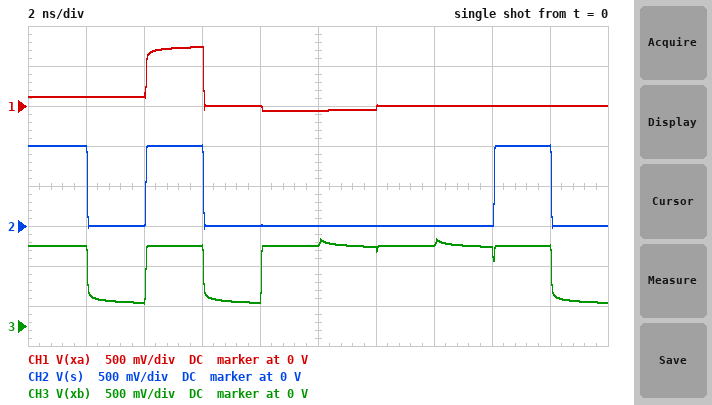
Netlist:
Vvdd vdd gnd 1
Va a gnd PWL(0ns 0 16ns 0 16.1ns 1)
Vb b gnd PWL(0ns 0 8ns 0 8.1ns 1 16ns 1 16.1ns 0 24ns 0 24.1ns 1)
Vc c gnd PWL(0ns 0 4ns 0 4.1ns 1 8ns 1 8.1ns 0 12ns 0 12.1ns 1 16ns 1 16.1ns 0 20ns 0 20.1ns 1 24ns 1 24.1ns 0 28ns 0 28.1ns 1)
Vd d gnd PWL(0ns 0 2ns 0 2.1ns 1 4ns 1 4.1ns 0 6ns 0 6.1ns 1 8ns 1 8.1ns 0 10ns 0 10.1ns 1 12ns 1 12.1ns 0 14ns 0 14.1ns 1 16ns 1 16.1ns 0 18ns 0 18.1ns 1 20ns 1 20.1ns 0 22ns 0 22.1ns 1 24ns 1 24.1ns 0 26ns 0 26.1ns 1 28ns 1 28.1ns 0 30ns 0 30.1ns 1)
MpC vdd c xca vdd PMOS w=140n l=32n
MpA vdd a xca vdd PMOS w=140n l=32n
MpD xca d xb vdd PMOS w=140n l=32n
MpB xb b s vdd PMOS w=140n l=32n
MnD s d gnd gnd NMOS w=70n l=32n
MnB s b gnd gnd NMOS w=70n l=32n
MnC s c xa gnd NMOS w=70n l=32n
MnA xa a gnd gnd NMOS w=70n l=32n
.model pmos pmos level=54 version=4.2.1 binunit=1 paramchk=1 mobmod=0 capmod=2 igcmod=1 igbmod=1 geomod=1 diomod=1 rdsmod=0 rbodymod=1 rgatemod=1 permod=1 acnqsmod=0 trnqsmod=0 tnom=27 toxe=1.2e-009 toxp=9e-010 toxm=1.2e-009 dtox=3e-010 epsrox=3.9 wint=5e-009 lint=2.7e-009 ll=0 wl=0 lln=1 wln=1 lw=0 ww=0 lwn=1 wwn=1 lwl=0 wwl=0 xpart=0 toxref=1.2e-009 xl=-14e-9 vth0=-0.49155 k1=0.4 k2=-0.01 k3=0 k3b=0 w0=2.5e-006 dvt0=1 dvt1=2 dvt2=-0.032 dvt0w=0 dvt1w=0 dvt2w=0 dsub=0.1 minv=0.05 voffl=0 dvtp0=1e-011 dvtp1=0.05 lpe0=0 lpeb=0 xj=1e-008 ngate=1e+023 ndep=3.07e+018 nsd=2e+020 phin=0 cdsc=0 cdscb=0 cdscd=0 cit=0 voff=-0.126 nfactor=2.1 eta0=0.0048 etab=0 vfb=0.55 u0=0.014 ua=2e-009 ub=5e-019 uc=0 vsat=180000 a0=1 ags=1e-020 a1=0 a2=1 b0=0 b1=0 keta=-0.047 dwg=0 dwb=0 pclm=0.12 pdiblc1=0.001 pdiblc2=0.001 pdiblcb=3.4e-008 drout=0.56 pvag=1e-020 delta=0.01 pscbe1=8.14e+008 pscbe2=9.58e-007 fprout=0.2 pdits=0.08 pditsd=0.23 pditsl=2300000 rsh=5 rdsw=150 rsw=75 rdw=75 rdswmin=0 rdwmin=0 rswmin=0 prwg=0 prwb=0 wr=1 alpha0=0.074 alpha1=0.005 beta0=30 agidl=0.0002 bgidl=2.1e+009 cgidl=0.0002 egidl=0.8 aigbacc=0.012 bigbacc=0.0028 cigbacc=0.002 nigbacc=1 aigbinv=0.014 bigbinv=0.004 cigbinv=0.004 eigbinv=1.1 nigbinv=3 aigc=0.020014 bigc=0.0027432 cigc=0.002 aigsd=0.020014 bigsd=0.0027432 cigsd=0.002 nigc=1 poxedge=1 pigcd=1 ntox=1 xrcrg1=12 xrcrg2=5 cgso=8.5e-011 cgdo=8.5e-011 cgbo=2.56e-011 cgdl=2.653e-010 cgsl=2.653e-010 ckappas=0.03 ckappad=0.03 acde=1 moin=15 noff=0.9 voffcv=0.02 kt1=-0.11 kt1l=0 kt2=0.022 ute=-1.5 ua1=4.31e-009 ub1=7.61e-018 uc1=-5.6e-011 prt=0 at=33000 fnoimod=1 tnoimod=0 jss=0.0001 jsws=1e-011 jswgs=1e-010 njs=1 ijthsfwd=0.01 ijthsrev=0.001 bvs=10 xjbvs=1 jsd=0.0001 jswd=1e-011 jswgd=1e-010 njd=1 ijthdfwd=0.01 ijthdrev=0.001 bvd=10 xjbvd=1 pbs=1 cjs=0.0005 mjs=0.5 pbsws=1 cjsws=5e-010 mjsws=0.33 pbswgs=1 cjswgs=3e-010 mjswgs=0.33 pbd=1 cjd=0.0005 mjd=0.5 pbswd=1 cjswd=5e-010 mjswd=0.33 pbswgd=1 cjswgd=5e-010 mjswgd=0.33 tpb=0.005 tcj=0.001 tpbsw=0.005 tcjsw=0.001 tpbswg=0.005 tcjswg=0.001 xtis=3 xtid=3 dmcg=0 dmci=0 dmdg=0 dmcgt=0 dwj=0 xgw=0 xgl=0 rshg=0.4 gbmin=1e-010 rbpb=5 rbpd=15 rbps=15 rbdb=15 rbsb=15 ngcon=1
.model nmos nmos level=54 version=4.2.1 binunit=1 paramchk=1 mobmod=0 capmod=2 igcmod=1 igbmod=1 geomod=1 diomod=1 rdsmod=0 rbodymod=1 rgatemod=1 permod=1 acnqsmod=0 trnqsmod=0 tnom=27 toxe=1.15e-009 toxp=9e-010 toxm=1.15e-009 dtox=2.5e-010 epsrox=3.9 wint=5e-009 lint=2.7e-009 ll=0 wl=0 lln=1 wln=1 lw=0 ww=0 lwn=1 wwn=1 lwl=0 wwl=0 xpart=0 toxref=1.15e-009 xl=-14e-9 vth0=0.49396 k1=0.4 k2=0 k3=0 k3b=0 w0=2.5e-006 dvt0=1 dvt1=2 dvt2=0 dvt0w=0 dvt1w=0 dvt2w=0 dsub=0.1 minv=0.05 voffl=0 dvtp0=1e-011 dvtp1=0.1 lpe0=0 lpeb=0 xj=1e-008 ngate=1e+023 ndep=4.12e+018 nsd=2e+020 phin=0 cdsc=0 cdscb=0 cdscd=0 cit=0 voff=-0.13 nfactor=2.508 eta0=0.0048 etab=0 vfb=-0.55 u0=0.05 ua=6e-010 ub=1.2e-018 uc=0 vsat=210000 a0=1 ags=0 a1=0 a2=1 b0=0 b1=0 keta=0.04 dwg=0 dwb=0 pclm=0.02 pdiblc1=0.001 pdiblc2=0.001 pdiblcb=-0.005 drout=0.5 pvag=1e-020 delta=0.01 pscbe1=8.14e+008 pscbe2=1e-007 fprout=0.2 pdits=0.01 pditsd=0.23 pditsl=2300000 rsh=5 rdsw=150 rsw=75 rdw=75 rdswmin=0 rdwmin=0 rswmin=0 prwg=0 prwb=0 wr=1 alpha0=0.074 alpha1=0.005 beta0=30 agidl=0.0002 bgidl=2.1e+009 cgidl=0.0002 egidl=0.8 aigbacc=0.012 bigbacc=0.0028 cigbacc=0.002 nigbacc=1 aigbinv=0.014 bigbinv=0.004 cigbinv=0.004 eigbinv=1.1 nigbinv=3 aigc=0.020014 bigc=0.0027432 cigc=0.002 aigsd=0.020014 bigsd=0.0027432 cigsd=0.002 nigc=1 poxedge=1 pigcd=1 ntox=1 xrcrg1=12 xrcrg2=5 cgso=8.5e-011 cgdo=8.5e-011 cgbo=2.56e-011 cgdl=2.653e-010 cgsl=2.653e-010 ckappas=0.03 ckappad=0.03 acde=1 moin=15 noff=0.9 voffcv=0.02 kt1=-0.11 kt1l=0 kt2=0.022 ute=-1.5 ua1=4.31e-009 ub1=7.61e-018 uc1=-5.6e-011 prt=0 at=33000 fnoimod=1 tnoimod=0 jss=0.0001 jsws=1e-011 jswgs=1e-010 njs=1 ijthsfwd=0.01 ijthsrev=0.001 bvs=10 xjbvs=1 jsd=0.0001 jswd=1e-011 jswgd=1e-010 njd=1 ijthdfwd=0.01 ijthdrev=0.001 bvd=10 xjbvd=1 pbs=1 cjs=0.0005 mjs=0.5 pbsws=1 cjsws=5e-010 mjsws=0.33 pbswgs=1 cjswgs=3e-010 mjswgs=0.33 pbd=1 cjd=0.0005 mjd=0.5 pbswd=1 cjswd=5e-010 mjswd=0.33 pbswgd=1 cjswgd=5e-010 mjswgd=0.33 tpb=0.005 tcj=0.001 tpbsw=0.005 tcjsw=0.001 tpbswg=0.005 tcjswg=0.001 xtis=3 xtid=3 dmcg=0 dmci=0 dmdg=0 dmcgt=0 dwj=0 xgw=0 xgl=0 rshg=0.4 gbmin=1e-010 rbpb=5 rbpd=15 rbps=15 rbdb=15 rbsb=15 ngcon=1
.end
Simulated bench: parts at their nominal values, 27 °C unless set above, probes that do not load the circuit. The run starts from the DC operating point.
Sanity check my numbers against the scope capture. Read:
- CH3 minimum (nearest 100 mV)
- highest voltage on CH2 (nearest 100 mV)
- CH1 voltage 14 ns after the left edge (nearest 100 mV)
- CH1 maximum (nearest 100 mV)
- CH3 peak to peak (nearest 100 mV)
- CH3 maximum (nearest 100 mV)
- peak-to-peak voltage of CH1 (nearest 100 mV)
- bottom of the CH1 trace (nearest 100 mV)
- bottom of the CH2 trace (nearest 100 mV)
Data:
300 mV
1.0 V
0 V
700 mV
800 mV
1.1 V
800 mV
-100 mV
0 V
